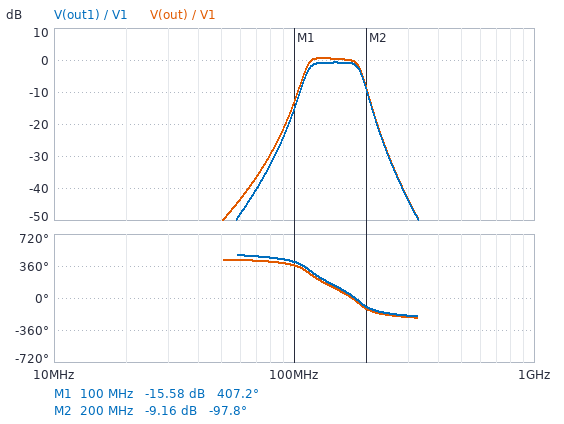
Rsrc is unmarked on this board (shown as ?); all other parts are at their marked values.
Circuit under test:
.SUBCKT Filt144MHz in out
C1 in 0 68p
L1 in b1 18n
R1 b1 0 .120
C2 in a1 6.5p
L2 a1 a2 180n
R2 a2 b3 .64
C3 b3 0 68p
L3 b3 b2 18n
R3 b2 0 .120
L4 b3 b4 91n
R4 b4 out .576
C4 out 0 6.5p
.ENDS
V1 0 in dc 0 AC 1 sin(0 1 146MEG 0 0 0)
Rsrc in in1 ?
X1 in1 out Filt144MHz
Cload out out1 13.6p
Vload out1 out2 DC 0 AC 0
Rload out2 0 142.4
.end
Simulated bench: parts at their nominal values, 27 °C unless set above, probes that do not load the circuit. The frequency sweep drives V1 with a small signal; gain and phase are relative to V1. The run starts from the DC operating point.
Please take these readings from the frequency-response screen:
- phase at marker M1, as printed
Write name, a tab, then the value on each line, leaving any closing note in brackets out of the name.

phase at marker M1, as printed	407.2 deg
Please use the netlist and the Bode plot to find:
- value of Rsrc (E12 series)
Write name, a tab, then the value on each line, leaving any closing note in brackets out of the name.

value of Rsrc	39 Ω
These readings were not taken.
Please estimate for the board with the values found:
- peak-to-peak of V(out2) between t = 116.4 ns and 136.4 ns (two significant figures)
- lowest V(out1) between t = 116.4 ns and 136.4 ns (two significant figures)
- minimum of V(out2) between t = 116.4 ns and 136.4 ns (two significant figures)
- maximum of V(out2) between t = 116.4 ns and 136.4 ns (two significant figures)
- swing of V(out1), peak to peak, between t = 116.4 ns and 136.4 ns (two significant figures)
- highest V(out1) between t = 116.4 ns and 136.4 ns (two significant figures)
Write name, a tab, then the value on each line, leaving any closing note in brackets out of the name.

peak-to-peak of V(out2) between t = 116.4 ns and 136.4 ns	1.8 V
lowest V(out1) between t = 116.4 ns and 136.4 ns	-910 mV
minimum of V(out2) between t = 116.4 ns and 136.4 ns	-910 mV
maximum of V(out2) between t = 116.4 ns and 136.4 ns	910 mV
swing of V(out1), peak to peak, between t = 116.4 ns and 136.4 ns	1.8 V
highest V(out1) between t = 116.4 ns and 136.4 ns	910 mV
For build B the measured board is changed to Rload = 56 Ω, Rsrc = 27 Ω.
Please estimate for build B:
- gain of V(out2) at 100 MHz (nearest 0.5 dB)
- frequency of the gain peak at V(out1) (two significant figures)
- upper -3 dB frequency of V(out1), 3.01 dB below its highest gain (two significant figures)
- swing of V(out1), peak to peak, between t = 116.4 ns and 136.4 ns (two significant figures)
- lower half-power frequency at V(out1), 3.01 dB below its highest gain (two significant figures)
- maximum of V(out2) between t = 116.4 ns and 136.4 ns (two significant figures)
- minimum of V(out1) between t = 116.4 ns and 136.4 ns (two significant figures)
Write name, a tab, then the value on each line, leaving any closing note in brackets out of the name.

gain of V(out2) at 100 MHz	-14.0 dB
frequency of the gain peak at V(out1)	140 MHz
upper -3 dB frequency of V(out1), 3.01 dB below its highest gain	190 MHz
swing of V(out1), peak to peak, between t = 116.4 ns and 136.4 ns	1.3 V
lower half-power frequency at V(out1), 3.01 dB below its highest gain	120 MHz
maximum of V(out2) between t = 116.4 ns and 136.4 ns	650 mV
minimum of V(out1) between t = 116.4 ns and 136.4 ns	-650 mV
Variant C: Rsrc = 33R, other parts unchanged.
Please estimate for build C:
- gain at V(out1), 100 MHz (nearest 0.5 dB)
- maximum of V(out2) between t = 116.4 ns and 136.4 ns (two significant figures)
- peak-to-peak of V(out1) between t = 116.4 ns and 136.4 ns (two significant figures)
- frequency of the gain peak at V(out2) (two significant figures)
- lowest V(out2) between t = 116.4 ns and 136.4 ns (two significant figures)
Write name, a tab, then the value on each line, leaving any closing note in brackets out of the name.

gain at V(out1), 100 MHz	-14.5 dB
maximum of V(out2) between t = 116.4 ns and 136.4 ns	980 mV
peak-to-peak of V(out1) between t = 116.4 ns and 136.4 ns	2.0 V
frequency of the gain peak at V(out2)	150 MHz
lowest V(out2) between t = 116.4 ns and 136.4 ns	-980 mV
